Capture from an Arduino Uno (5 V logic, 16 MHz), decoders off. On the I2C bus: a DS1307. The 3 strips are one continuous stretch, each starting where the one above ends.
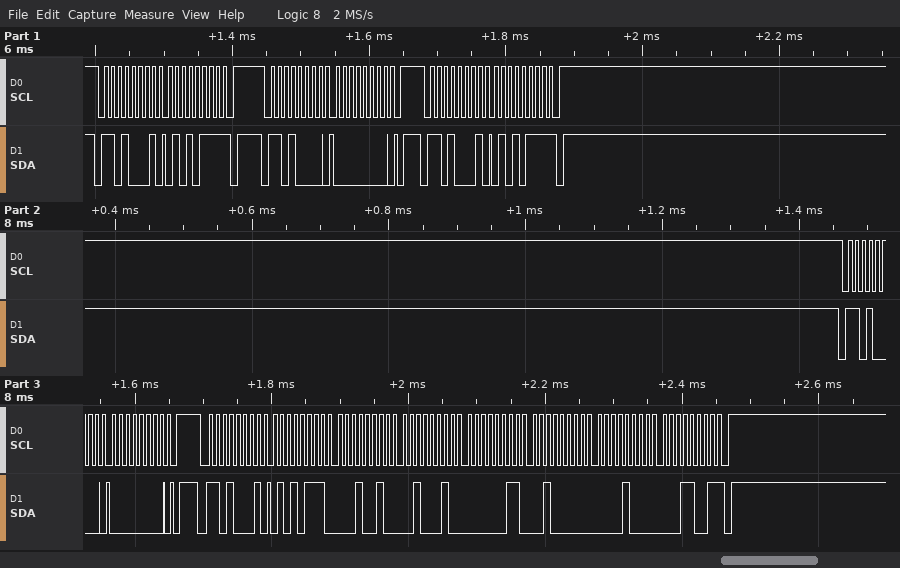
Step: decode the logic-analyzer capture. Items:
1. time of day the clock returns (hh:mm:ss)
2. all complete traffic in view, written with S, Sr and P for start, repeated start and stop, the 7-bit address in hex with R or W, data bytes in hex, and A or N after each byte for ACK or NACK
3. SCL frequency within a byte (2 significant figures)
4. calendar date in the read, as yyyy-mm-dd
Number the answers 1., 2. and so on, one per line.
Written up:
1. 22:12:57
2. S 68R A 57 N P S 68W A 00 A P S 68R A 57 N P S 68W A 00 A P S 68R A 57 A 12 A 22 A 03 A 20 A 08 A 19 N P
3. 100 kHz
4. 2019-08-20
